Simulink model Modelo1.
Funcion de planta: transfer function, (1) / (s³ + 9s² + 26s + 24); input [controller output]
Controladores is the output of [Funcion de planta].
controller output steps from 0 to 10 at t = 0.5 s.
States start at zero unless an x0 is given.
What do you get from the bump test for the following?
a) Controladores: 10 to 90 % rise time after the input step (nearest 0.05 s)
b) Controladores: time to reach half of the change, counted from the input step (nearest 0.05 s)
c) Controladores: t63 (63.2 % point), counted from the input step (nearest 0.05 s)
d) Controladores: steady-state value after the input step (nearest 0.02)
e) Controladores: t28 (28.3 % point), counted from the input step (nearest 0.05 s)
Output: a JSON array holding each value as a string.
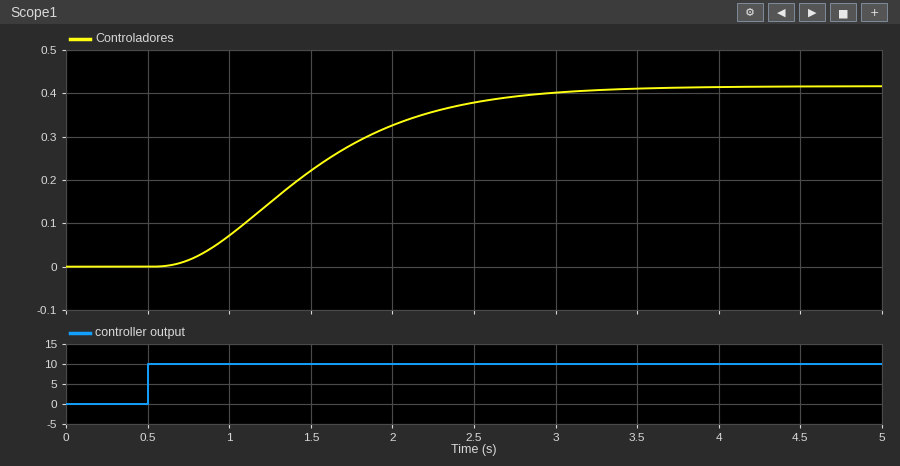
["1.55 s", "0.95 s", "1.15 s", "0.42", "0.65 s"]
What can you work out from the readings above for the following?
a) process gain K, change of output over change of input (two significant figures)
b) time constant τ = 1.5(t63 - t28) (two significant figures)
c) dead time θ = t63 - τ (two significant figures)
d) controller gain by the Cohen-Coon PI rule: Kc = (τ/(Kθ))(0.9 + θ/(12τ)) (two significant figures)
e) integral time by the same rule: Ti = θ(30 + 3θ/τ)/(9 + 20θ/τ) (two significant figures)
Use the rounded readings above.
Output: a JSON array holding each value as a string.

["0.042", "0.75 s", "0.40 s", "42", "0.64 s"]
